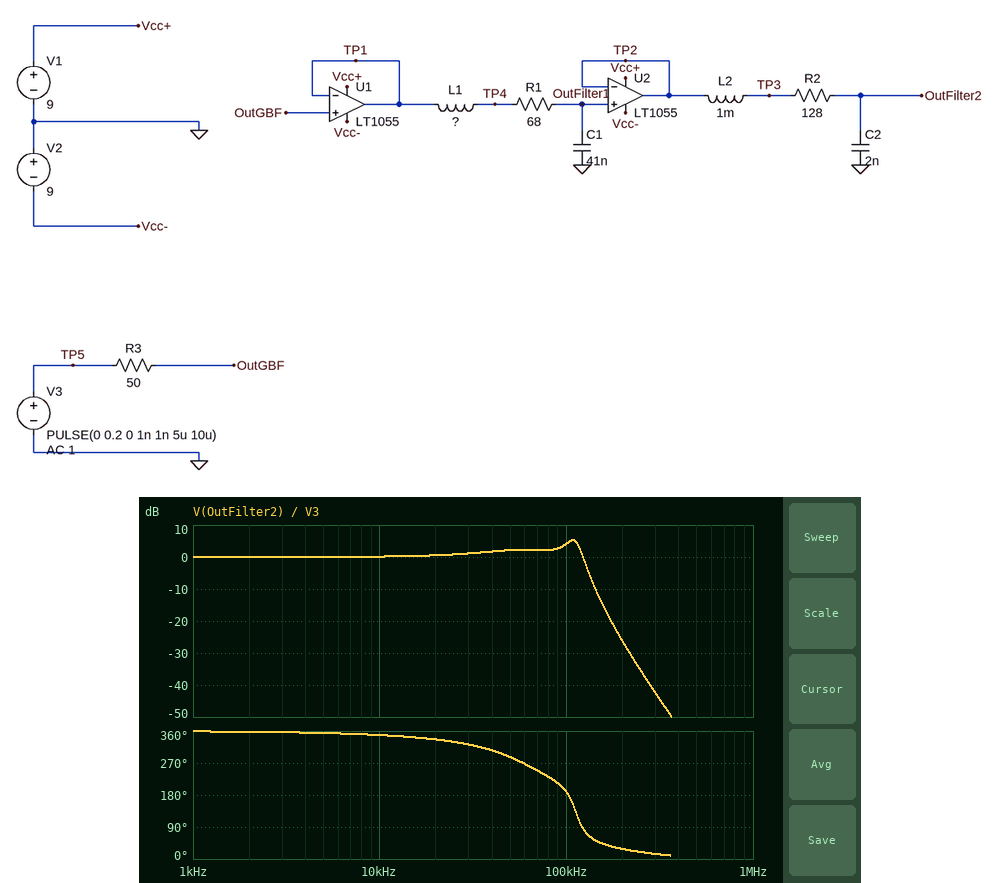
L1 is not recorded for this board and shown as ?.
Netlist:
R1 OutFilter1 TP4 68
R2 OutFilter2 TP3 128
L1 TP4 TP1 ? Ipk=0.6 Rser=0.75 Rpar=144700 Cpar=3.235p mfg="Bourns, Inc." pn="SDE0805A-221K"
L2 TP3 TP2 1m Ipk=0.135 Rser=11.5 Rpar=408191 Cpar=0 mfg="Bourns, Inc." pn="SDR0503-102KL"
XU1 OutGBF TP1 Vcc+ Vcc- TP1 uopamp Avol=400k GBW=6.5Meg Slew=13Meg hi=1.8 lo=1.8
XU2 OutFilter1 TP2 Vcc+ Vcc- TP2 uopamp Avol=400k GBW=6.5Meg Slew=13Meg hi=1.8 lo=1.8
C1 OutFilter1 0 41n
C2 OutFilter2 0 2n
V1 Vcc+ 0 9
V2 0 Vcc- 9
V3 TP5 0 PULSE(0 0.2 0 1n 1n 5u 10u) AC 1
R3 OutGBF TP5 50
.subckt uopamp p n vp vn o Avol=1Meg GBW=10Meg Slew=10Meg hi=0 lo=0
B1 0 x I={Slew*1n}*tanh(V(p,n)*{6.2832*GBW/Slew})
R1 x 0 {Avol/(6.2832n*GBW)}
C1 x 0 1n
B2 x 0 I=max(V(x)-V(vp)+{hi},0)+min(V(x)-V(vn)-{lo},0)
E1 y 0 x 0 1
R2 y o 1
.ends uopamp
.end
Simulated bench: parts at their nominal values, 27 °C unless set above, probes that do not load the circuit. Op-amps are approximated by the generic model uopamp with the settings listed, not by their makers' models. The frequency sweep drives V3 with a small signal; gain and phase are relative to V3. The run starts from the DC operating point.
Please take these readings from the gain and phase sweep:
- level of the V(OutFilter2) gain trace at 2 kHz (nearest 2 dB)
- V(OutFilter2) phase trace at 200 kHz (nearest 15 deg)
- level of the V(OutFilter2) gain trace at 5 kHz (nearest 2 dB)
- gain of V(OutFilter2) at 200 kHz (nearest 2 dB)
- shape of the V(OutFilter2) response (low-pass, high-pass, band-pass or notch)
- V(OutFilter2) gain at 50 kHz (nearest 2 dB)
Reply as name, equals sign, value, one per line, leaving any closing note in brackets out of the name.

level of the V(OutFilter2) gain trace at 2 kHz = 0 dB
V(OutFilter2) phase trace at 200 kHz = 30 deg
level of the V(OutFilter2) gain trace at 5 kHz = 0 dB
gain of V(OutFilter2) at 200 kHz = -26 dB
shape of the V(OutFilter2) response = low-pass
V(OutFilter2) gain at 50 kHz = 2 dB
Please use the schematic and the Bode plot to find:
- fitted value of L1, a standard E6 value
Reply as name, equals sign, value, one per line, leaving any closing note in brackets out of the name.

fitted value of L1, a standard E6 value = 150 µH
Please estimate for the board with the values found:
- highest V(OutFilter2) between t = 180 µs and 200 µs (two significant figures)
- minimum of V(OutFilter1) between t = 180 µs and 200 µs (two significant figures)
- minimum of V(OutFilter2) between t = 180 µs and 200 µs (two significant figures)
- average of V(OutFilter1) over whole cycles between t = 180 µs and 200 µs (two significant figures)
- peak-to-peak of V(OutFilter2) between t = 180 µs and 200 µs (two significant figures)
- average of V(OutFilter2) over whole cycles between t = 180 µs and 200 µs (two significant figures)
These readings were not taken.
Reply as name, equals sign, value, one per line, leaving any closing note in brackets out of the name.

highest V(OutFilter2) between t = 180 µs and 200 µs = 300 mV
minimum of V(OutFilter1) between t = 180 µs and 200 µs = 43 mV
minimum of V(OutFilter2) between t = 180 µs and 200 µs = -100 mV
average of V(OutFilter1) over whole cycles between t = 180 µs and 200 µs = 100 mV
peak-to-peak of V(OutFilter2) between t = 180 µs and 200 µs = 410 mV
average of V(OutFilter2) over whole cycles between t = 180 µs and 200 µs = 100 mV
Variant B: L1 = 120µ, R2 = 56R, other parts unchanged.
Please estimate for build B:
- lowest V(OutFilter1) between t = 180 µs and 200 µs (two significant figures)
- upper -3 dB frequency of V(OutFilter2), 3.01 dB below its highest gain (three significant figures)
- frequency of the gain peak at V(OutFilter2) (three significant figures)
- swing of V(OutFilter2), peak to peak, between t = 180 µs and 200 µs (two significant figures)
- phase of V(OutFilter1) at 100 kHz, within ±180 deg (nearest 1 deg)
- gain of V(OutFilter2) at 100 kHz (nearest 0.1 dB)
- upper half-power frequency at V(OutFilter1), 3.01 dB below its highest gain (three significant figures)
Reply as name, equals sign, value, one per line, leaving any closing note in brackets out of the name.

lowest V(OutFilter1) between t = 180 µs and 200 µs = 34 mV
upper -3 dB frequency of V(OutFilter2), 3.01 dB below its highest gain = 117 kHz
frequency of the gain peak at V(OutFilter2) = 112 kHz
swing of V(OutFilter2), peak to peak, between t = 180 µs and 200 µs = 560 mV
phase of V(OutFilter1) at 100 kHz, within ±180 deg = -119 deg
gain of V(OutFilter2) at 100 kHz = 6.8 dB
upper half-power frequency at V(OutFilter1), 3.01 dB below its highest gain = 77.7 kHz
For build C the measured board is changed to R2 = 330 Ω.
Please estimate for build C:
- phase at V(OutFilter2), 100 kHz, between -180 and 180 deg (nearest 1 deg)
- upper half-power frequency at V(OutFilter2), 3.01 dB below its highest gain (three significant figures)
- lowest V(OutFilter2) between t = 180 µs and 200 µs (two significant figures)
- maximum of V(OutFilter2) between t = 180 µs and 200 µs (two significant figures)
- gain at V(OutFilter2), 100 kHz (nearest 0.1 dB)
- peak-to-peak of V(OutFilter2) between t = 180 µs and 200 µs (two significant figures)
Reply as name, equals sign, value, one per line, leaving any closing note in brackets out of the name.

phase at V(OutFilter2), 100 kHz, between -180 and 180 deg = 165 deg
upper half-power frequency at V(OutFilter2), 3.01 dB below its highest gain = 103 kHz
lowest V(OutFilter2) between t = 180 µs and 200 µs = -17 mV
maximum of V(OutFilter2) between t = 180 µs and 200 µs = 220 mV
gain at V(OutFilter2), 100 kHz = -0.8 dB
peak-to-peak of V(OutFilter2) between t = 180 µs and 200 µs = 230 mV
